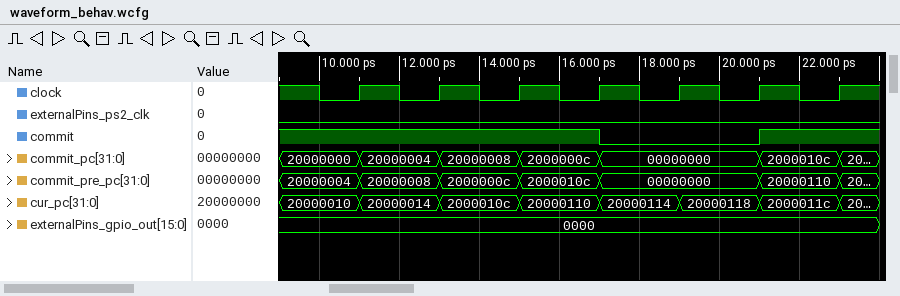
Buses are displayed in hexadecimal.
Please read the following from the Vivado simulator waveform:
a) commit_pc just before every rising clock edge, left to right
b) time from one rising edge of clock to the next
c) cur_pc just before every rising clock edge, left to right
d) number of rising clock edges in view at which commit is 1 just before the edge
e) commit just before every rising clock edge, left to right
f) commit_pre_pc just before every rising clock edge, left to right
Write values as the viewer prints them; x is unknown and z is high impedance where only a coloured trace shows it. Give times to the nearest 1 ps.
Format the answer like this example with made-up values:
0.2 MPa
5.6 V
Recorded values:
20000000, 20000004, 20000008, 2000000c, 00000000, 00000000, 2000010c
2 ps
20000010, 20000014, 2000010c, 20000110, 20000114, 20000118, 2000011c
5
1 1 1 1 0 0 1
20000004, 20000008, 2000000c, 2000010c, 00000000, 00000000, 20000110
